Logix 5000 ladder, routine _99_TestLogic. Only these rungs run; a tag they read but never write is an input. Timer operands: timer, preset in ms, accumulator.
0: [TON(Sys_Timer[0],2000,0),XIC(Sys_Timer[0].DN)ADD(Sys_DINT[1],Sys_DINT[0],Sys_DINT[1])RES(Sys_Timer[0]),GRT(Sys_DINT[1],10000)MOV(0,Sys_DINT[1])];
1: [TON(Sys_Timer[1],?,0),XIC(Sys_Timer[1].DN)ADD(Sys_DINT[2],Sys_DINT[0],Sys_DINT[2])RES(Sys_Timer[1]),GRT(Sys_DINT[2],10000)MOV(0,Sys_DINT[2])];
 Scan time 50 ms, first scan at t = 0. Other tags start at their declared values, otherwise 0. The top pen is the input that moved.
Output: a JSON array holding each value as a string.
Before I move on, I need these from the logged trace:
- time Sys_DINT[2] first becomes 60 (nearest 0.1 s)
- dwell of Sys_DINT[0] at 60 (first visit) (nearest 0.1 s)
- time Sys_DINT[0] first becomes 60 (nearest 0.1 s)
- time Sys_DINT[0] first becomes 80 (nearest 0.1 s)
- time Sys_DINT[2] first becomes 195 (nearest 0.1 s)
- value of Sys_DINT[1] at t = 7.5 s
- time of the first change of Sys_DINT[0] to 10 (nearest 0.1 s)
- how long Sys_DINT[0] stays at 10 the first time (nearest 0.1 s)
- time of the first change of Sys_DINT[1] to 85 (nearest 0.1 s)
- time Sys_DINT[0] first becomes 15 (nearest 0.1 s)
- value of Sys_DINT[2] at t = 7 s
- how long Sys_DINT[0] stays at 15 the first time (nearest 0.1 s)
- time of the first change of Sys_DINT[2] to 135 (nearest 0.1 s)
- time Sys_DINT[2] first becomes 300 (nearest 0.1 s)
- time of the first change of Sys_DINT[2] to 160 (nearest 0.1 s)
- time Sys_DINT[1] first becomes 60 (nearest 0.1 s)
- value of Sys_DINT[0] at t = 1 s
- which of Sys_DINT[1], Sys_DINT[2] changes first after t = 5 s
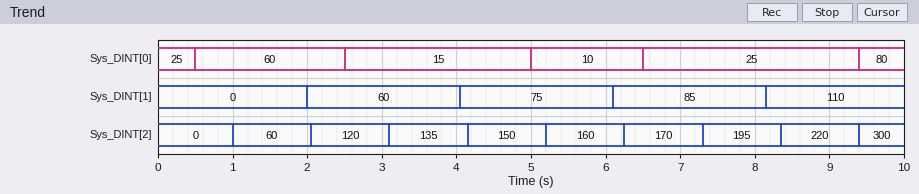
["1.0 s", "2.0 s", "0.5 s", "9.4 s", "7.3 s", "85", "5.0 s", "1.5 s", "6.1 s", "2.5 s", "170", "2.5 s", "3.1 s", "9.4 s", "5.2 s", "2.0 s", "60", "Sys_DINT[2]"]
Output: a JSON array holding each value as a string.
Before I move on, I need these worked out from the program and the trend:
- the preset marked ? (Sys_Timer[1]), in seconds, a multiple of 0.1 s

["1.0 s"]
